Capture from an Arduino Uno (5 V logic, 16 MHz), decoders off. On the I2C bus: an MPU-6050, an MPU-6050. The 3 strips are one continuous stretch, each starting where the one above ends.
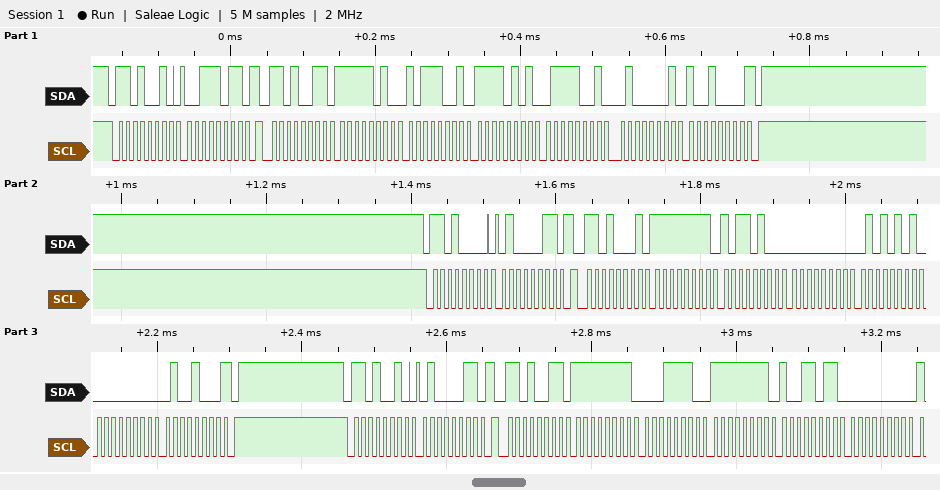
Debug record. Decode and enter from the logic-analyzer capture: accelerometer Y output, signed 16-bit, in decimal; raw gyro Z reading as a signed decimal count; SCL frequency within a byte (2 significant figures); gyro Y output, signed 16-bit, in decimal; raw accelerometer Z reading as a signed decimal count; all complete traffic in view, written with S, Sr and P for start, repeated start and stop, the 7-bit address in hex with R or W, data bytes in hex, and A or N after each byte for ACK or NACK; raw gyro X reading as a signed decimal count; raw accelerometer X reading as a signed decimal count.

-2695
72
100 kHz
85
16784
S 69W A 3B A Sr 69R A FA A B9 A F5 A 79 A 41 A 90 N P S 68W A 43 A Sr 68R A FF A B4 A 00 A 55 A 00 A 48 N P S 69W A 43 A Sr 69R A FF A 1E A FF A 9B A 00 A
-76
-1351
